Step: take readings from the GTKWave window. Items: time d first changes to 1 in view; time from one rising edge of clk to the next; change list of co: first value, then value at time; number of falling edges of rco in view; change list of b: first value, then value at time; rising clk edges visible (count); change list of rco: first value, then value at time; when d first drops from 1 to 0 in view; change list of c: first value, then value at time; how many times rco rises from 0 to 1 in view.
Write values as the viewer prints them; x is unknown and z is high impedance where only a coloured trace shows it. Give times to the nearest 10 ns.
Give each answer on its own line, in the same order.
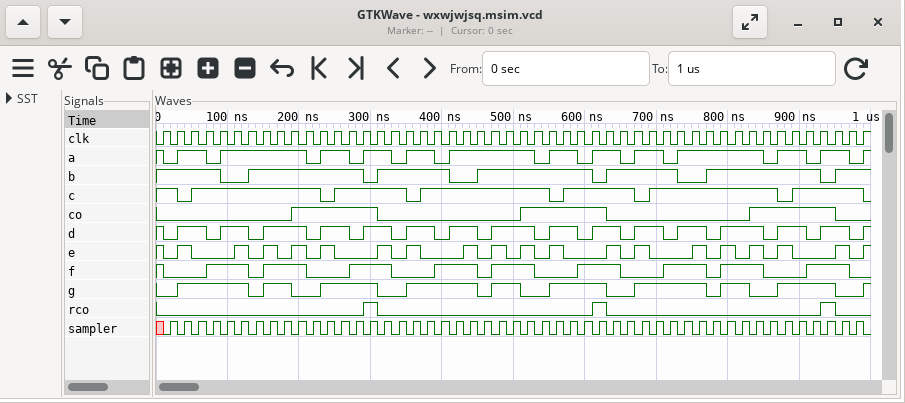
30 ns
20 ns
0, 1 at 190 ns, 0 at 310 ns, 1 at 510 ns, 0 at 630 ns, 1 at 830 ns, 0 at 950 ns
3
1, 0 at 90 ns, 1 at 130 ns, 0 at 290 ns, 1 at 310 ns, 0 at 410 ns, 1 at 450 ns, 0 at 610 ns, 1 at 630 ns, 0 at 730 ns, 1 at 770 ns, 0 at 930 ns, 1 at 950 ns
50
0, 1 at 290 ns, 0 at 310 ns, 1 at 610 ns, 0 at 630 ns, 1 at 930 ns, 0 at 950 ns
10 ns
1, 0 at 30 ns, 1 at 50 ns, 0 at 230 ns, 1 at 250 ns, 0 at 350 ns, 1 at 370 ns, 0 at 550 ns, 1 at 570 ns, 0 at 670 ns, 1 at 690 ns, 0 at 870 ns, 1 at 890 ns, 0 at 990 ns
3
